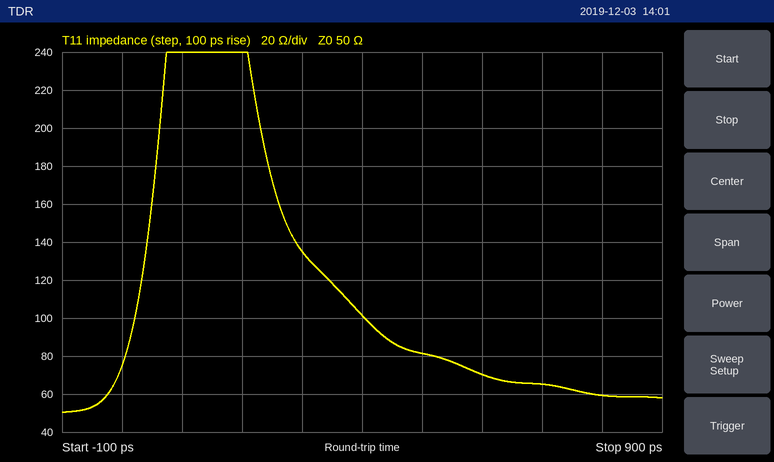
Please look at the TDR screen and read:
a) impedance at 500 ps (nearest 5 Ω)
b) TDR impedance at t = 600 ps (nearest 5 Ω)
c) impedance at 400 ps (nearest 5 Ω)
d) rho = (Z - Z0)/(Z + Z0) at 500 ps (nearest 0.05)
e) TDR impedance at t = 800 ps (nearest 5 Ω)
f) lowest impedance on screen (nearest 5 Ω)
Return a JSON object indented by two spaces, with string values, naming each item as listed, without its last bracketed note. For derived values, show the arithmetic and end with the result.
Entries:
{
  "impedance at 500 ps": "80 Ω",
  "TDR impedance at t = 600 ps": "70 Ω",
  "impedance at 400 ps": "100 Ω",
  "rho = (Z - Z0)/(Z + Z0) at 500 ps": "(80 − 50)/(80 + 50) ≈ +0.231, so +0.25 to the nearest 0.05",
  "TDR impedance at t = 800 ps": "60 Ω",
  "lowest impedance on screen": "50 Ω"
}
